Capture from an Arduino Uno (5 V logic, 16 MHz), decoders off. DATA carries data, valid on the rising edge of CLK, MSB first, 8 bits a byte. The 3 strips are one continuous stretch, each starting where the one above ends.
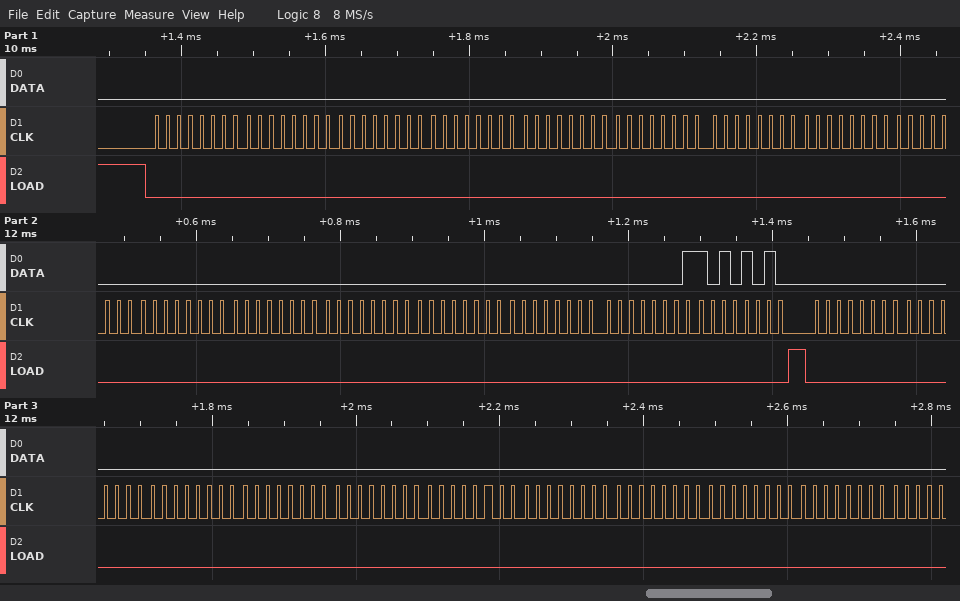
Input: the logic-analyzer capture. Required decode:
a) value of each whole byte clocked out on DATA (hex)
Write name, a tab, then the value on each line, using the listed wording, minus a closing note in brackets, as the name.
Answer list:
value of each whole byte clocked out on DATA	00 00 00 00 00 00 00 00 00 00 00 00 00 00 01 AA 00 00 00 00 00 00 00 00 00 00
